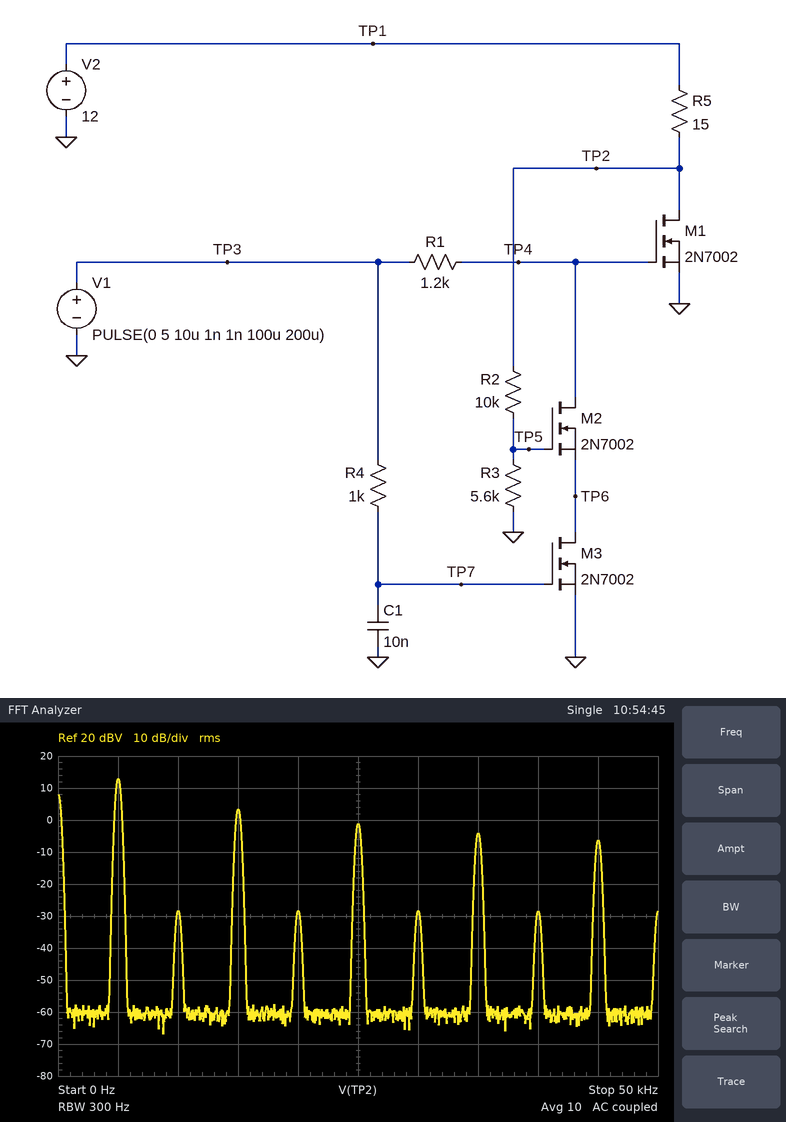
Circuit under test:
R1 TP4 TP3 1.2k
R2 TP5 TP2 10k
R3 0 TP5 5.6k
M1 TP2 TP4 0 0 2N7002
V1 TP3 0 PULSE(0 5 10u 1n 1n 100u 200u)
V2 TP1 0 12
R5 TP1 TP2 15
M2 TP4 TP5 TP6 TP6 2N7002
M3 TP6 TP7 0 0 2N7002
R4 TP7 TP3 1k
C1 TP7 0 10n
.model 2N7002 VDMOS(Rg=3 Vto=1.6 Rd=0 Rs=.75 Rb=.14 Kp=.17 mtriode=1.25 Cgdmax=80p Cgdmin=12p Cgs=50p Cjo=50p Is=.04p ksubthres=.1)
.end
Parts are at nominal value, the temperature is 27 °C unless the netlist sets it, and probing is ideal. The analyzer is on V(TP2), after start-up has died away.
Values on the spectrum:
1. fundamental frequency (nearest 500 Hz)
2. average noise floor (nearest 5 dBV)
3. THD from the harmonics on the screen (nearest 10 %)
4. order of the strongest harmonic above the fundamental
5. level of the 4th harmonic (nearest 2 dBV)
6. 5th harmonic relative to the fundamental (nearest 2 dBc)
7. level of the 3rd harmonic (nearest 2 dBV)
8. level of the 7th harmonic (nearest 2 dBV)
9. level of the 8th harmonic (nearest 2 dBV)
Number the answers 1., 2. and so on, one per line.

1. 5.0 kHz
2. -60 dBV
3. 40 %
4. 3
5. -28 dBV
6. -14 dBc
7. 4 dBV
8. -4 dBV
9. -28 dBV
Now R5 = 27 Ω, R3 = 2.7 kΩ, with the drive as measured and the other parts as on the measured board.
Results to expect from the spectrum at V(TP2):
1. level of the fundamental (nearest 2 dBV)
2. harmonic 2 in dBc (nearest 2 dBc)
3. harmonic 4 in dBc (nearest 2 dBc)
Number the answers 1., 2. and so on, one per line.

1. 14 dBV
2. -50 dBc
3. -50 dBc
